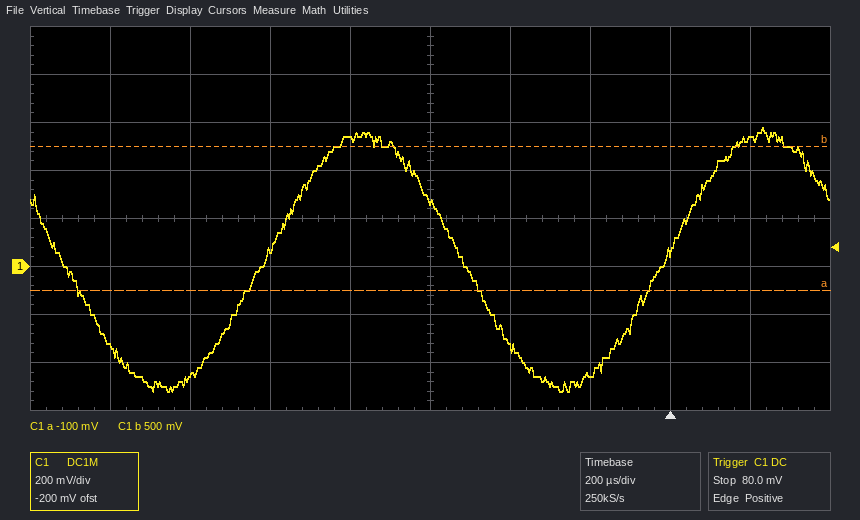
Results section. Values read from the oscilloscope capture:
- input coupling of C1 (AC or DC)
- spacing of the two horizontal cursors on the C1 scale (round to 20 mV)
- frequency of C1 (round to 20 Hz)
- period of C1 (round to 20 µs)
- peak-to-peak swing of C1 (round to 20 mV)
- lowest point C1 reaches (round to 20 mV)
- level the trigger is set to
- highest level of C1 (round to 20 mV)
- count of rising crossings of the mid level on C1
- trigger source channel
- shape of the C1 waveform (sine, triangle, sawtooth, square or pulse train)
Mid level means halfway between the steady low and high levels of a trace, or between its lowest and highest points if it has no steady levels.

DC
600 mV
1.00 kHz
1.00 ms
1.10 V
-520 mV
80.0 mV
580 mV
2
C1
sine
